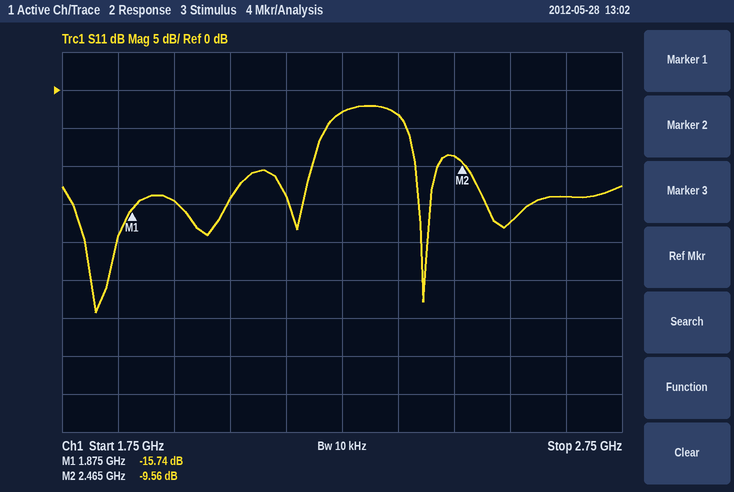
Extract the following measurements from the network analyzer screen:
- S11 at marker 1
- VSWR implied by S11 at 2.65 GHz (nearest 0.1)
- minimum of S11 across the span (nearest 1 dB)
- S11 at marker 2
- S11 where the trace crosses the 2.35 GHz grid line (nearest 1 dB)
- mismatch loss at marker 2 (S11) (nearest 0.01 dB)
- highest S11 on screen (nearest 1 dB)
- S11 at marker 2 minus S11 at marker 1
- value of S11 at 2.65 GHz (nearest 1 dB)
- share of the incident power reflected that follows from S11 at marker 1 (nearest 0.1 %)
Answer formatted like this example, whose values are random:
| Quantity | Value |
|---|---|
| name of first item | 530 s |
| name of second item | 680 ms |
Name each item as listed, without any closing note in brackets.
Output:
| Quantity | Value |
|---|---|
| S11 at marker 1 | -15.74 dB |
| VSWR implied by S11 at 2.65 GHz | 1.5 |
| minimum of S11 across the span | -29 dB |
| S11 at marker 2 | -9.56 dB |
| S11 where the trace crosses the 2.35 GHz grid line | -3 dB |
| mismatch loss at marker 2 (S11) | 0.51 dB |
| highest S11 on screen | -2 dB |
| S11 at marker 2 minus S11 at marker 1 | 6.18 dB |
| value of S11 at 2.65 GHz | -14 dB |
| share of the incident power reflected that follows from S11 at marker 1 | 2.7 % |
